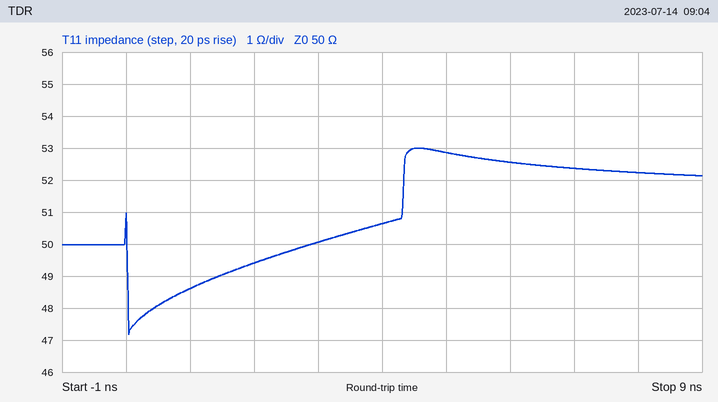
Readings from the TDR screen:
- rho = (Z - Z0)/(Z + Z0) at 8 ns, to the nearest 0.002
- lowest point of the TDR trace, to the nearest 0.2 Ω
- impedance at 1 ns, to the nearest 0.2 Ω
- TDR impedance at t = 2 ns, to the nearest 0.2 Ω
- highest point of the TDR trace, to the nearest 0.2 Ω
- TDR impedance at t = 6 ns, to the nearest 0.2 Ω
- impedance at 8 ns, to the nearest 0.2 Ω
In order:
+0.022
47.2 Ω
48.6 Ω
49.4 Ω
53.0 Ω
52.6 Ω
52.2 Ω
